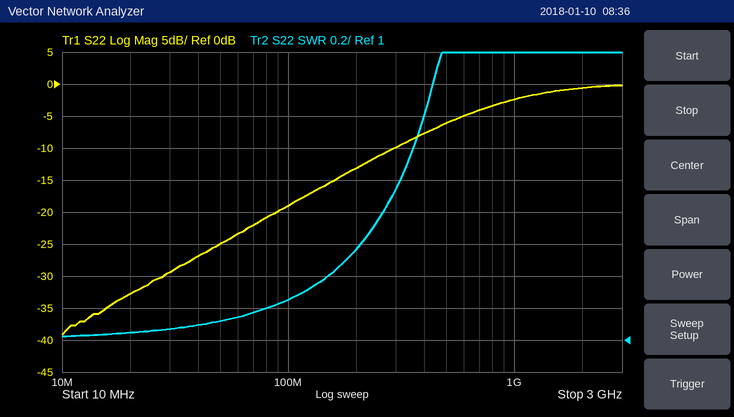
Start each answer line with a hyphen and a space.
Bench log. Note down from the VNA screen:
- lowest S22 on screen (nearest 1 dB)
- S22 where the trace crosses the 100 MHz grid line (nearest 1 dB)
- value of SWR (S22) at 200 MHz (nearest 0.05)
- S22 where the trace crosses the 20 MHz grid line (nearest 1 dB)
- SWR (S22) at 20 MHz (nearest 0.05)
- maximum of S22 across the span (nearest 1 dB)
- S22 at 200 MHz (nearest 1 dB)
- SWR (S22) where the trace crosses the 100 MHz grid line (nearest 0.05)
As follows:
- -39 dB
- -19 dB
- 1.55
- -33 dB
- 1.05
- 0 dB
- -13 dB
- 1.25
